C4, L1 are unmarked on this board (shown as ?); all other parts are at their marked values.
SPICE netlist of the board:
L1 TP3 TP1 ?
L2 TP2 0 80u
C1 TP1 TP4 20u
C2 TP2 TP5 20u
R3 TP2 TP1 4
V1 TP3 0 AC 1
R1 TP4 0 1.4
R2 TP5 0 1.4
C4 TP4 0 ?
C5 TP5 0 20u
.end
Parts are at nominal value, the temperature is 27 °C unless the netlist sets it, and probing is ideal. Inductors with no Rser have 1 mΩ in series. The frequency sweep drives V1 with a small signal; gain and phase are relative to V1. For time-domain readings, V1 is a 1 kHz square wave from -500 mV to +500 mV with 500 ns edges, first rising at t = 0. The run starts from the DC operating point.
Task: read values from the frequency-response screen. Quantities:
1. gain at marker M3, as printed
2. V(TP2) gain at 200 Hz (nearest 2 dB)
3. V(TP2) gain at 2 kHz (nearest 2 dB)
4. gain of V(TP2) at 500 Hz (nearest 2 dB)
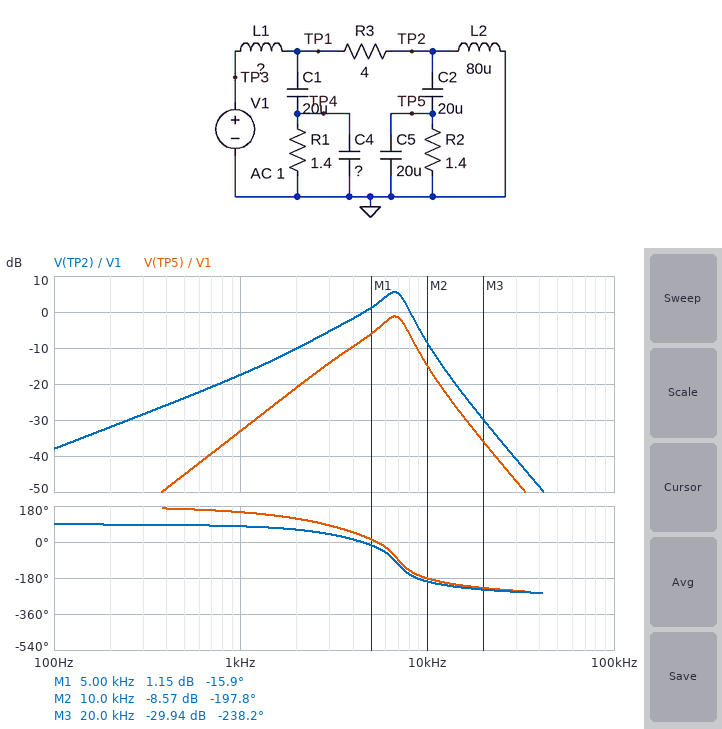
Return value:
-29.94 dB
-32 dB
-10 dB
-24 dB
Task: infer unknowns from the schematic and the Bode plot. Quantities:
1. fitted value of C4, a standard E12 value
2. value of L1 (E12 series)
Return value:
39 µF
33 µH
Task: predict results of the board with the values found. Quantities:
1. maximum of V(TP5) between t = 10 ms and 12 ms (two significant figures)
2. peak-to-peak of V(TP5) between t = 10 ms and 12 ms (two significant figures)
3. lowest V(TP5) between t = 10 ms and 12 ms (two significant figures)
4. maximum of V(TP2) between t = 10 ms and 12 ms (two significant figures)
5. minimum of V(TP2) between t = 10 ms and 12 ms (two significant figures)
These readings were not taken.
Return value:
190 mV
390 mV
-190 mV
520 mV
-520 mV
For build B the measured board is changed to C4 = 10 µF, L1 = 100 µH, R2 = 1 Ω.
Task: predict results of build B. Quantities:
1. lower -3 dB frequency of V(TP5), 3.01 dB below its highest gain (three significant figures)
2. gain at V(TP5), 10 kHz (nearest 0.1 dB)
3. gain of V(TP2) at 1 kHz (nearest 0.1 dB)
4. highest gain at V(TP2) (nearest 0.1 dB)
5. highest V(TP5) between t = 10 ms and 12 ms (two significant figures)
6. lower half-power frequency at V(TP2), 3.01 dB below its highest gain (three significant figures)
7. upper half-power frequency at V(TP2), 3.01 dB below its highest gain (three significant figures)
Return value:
3.29 kHz
-27.6 dB
-17.2 dB
-1.3 dB
76 mV
3.02 kHz
5.10 kHz
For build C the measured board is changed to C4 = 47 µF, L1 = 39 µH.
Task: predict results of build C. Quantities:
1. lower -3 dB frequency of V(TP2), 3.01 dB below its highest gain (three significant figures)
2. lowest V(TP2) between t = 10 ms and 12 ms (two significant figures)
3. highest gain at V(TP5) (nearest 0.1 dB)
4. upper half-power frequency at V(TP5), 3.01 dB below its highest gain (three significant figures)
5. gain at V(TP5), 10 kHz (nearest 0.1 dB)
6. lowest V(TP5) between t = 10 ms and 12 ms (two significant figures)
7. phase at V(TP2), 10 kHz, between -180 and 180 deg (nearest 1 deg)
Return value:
5.28 kHz
-470 mV
0.1 dB
6.90 kHz
-17.9 dB
-180 mV
155 deg
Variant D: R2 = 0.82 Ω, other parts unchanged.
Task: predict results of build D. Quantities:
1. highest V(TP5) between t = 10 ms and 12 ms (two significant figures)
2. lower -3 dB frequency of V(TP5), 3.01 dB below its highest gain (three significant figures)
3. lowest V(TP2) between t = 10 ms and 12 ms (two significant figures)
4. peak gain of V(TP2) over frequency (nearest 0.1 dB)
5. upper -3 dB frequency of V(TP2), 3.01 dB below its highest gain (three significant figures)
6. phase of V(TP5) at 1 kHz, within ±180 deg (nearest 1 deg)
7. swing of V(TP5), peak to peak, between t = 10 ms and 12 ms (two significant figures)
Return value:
150 mV
5.12 kHz
-490 mV
3.3 dB
7.66 kHz
157 deg
290 mV
